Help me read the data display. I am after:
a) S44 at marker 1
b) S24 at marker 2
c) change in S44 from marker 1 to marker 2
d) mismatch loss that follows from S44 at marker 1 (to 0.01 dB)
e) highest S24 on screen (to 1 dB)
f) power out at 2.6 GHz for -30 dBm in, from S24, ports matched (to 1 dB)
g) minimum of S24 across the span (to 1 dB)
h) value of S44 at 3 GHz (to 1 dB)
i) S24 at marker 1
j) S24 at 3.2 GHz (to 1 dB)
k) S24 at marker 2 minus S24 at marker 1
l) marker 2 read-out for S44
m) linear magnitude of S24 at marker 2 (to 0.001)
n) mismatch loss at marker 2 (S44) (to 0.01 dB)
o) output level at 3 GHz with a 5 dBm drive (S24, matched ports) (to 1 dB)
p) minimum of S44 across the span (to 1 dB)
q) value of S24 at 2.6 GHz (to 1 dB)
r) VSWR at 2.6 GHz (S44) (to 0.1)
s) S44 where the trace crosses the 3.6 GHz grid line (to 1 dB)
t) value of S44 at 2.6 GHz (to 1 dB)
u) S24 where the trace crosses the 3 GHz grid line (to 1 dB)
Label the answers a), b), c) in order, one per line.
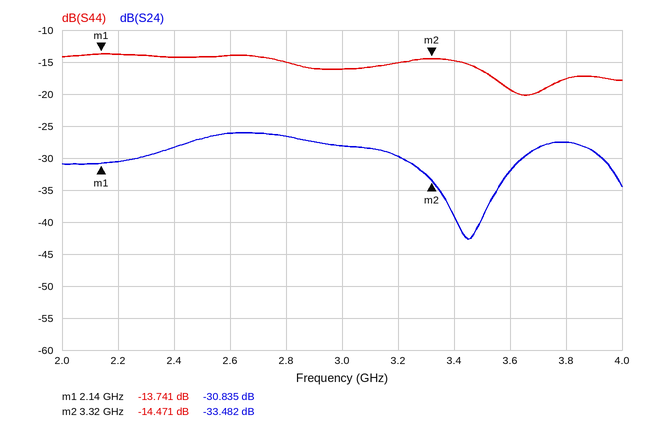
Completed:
a) -13.741 dB
b) -33.482 dB
c) -0.730 dB
d) 0.19 dB
e) -26 dB
f) -56 dBm
g) -43 dB
h) -16 dB
i) -30.835 dB
j) -30 dB
k) -2.647 dB
l) -14.471 dB
m) 0.021
n) 0.16 dB
o) -23 dBm
p) -20 dB
q) -26 dB
r) 1.5
s) -19 dB
t) -14 dB
u) -28 dB
